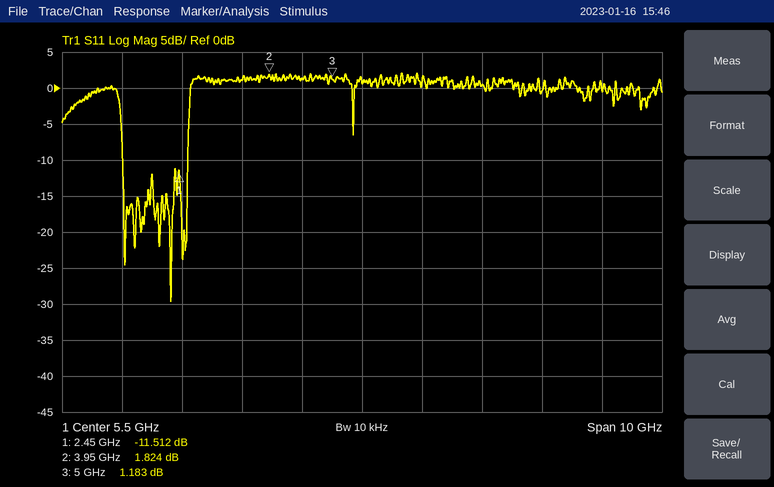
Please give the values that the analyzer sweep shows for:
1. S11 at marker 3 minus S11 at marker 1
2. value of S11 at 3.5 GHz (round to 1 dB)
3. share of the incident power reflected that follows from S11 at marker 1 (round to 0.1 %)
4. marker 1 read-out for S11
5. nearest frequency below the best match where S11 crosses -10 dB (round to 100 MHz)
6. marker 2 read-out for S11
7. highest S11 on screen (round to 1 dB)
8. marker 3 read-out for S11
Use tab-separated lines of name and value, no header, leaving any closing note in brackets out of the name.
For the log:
S11 at marker 3 minus S11 at marker 1	12.695 dB
value of S11 at 3.5 GHz	1 dB
share of the incident power reflected that follows from S11 at marker 1	7.1 %
marker 1 read-out for S11	-11.512 dB
nearest frequency below the best match where S11 crosses -10 dB	1.5 GHz
marker 2 read-out for S11	1.824 dB
highest S11 on screen	2 dB
marker 3 read-out for S11	1.183 dB
